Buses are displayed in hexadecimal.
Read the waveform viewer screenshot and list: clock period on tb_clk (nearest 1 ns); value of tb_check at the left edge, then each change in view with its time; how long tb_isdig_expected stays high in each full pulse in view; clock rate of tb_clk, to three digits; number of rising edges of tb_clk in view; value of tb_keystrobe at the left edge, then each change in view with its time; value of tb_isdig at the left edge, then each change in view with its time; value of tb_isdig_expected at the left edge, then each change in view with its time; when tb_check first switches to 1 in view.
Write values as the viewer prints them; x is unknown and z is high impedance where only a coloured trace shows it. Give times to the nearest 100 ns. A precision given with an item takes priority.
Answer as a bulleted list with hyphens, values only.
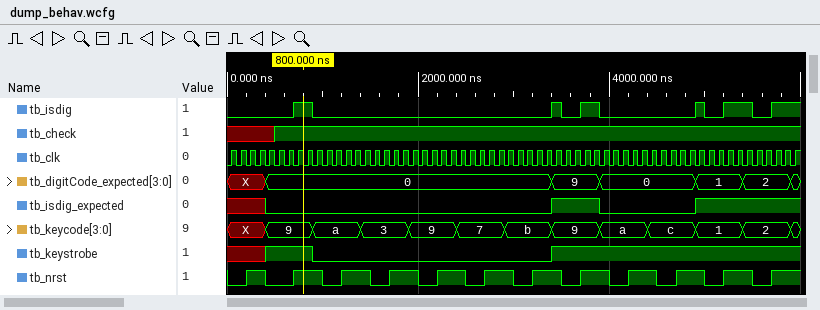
- 100 ns
- x, 1 at 500 ns
- 500 ns
- 10.0 MHz
- 60
- x, 1 at 400 ns, 0 at 900 ns, 1 at 3400 ns
- 0, 1 at 700 ns, 0 at 900 ns, 1 at 3400 ns, 0 at 3500 ns, 1 at 3700 ns, 0 at 3900 ns, 1 at 4900 ns, 0 at 5000 ns, 1 at 5200 ns, 0 at 5500 ns, 1 at 5700 ns
- x, 0 at 400 ns, 1 at 3400 ns, 0 at 3900 ns, 1 at 4900 ns
- 500 ns
